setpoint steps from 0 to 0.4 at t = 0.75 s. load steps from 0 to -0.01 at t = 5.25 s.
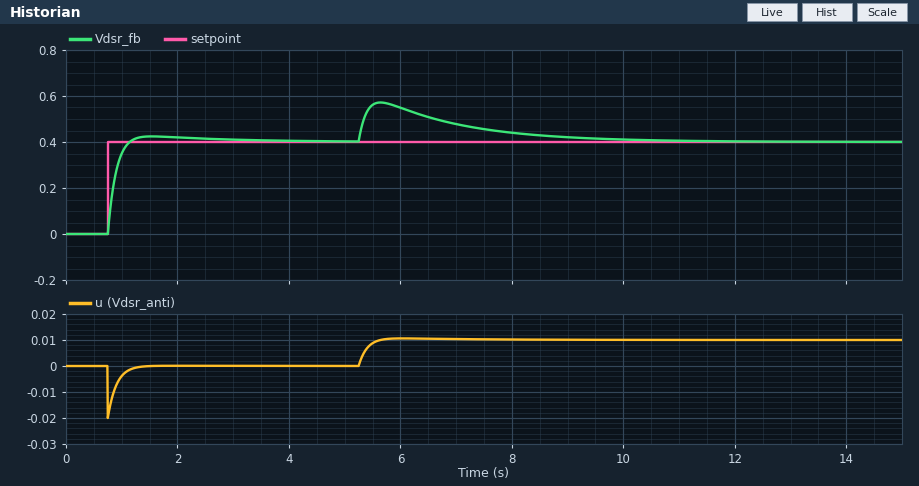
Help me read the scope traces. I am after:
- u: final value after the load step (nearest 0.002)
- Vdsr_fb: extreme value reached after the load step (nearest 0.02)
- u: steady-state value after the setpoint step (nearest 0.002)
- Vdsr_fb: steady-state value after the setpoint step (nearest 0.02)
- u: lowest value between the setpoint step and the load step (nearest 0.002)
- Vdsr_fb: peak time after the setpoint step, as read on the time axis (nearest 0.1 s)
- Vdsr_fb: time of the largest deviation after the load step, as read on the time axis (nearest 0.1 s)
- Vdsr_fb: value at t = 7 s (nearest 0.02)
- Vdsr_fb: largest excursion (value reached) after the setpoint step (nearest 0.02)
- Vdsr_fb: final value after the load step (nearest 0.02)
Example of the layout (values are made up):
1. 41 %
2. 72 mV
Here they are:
1. 0.010
2. 0.58
3. 0.000
4. 0.40
5. -0.020
6. 1.5 s
7. 5.6 s
8. 0.48
9. 0.42
10. 0.40
